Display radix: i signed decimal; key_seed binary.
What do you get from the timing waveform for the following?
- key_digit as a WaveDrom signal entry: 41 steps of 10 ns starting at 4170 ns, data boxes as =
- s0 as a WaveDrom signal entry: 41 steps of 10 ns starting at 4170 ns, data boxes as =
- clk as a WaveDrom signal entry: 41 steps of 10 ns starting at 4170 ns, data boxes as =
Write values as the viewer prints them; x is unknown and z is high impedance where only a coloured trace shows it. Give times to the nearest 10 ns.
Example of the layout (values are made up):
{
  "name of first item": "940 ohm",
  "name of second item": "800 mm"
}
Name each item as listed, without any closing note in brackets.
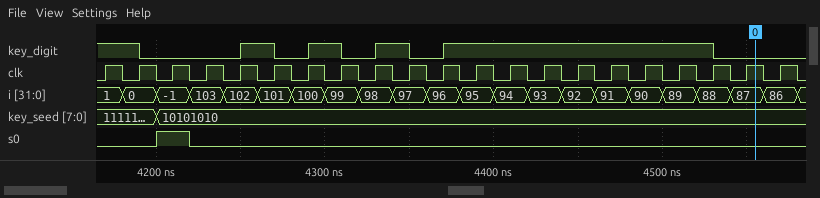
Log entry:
{
  "key_digit as a WaveDrom signal entry: 41 steps of 10 ns starting at 4170 ns, data boxes as =": "{name: 'key_digit', wave: '1.0.....1.0.1.0.1.0.1...............0....'}",
  "s0 as a WaveDrom signal entry: 41 steps of 10 ns starting at 4170 ns, data boxes as =": "{name: 's0', wave: '0..1.0...................................'}",
  "clk as a WaveDrom signal entry: 41 steps of 10 ns starting at 4170 ns, data boxes as =": "{name: 'clk', wave: '10101010101010101010101010101010101010101'}"
}
